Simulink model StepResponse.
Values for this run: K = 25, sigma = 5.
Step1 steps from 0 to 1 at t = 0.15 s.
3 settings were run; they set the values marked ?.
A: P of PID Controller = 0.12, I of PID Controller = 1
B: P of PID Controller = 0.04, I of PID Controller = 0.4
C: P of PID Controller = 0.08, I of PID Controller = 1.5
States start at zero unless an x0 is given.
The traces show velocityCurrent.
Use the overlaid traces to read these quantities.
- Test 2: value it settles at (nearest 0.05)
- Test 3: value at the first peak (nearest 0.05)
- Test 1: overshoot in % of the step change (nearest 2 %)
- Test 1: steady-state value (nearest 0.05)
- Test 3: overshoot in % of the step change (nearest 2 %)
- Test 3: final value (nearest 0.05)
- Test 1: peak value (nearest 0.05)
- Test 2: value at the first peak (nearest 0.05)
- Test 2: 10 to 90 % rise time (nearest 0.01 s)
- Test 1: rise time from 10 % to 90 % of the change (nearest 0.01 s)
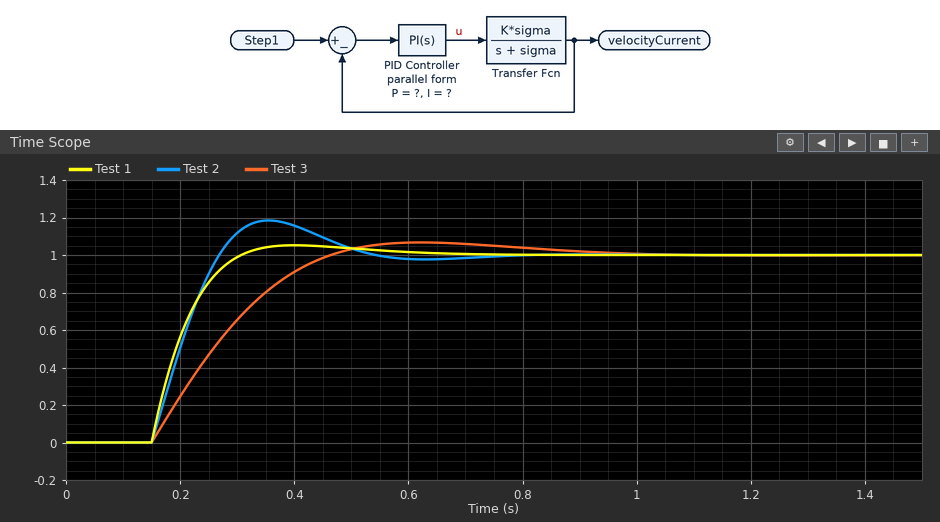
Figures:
1.00
1.05
6 %
1.00
6 %
1.00
1.05
1.20
0.09 s
0.11 s
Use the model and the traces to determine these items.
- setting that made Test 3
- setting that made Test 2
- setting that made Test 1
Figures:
B
C
A
